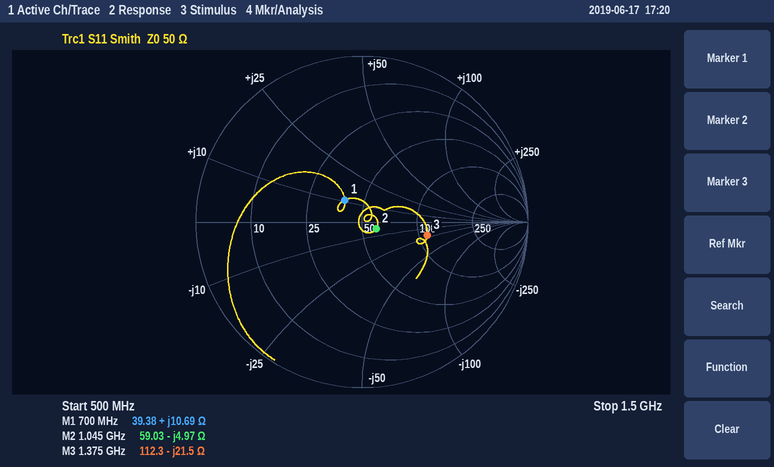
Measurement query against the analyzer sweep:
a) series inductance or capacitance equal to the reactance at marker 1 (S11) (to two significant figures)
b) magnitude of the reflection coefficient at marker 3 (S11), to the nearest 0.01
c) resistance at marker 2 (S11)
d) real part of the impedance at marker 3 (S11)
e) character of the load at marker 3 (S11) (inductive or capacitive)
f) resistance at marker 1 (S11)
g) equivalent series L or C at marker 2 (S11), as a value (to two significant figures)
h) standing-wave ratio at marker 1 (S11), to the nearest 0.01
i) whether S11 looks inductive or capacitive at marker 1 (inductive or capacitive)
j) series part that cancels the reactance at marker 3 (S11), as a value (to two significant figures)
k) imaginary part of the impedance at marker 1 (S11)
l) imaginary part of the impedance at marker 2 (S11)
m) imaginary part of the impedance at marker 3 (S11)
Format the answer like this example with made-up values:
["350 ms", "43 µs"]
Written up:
["2.4 nH", "0.40", "59.03 Ω", "112.3 Ω", "capacitive", "39.38 Ω", "31 pF", "1.40", "inductive", "2.5 nH", "+10.69 Ω", "-4.97 Ω", "-21.5 Ω"]
